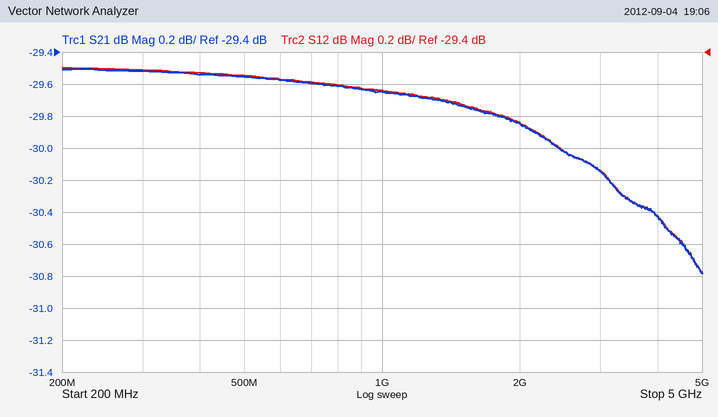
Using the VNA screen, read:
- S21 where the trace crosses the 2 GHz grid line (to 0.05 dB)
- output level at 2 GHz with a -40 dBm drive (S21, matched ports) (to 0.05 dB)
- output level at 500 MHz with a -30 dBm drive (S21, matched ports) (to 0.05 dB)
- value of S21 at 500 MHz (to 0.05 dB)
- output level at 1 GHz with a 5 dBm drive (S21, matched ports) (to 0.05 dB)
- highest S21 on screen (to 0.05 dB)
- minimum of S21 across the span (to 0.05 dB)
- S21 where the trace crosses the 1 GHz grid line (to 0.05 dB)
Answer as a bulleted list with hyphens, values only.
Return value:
- -29.85 dB
- -69.85 dBm
- -59.55 dBm
- -29.55 dB
- -24.65 dBm
- -29.50 dB
- -30.80 dB
- -29.65 dB
